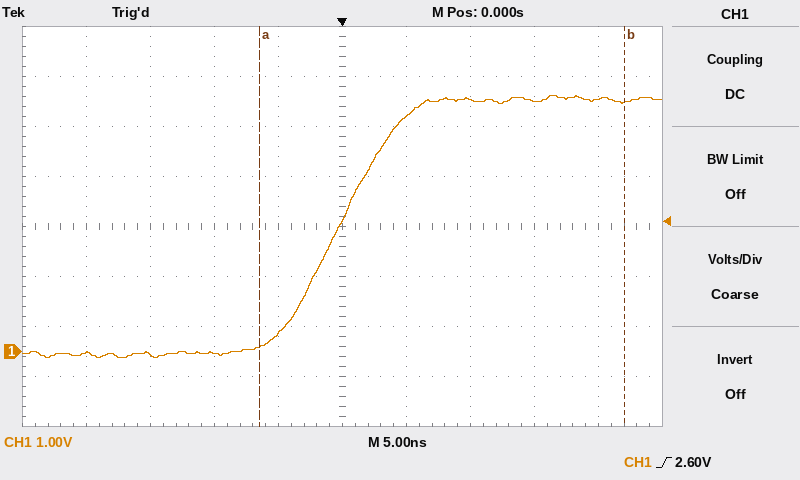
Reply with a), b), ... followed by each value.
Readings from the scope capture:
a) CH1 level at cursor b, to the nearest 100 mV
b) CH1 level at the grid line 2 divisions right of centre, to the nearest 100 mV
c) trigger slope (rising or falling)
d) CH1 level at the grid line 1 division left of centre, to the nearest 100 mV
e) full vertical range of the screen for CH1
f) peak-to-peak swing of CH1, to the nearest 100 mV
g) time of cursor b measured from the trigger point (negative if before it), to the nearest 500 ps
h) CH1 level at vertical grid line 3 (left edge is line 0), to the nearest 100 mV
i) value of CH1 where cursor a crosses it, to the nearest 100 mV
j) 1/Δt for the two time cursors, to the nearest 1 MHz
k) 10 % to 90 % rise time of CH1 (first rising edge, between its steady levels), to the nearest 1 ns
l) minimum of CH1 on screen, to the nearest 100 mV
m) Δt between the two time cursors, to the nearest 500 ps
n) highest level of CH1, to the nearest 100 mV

a) 5.0 V
b) 5.0 V
c) rising
d) 400 mV
e) 8 V
f) 5.2 V
g) +22.0 ns
h) 0.0 V
i) 100 mV
j) 35 MHz
k) 9 ns
l) -100 mV
m) 28.5 ns
n) 5.1 V
